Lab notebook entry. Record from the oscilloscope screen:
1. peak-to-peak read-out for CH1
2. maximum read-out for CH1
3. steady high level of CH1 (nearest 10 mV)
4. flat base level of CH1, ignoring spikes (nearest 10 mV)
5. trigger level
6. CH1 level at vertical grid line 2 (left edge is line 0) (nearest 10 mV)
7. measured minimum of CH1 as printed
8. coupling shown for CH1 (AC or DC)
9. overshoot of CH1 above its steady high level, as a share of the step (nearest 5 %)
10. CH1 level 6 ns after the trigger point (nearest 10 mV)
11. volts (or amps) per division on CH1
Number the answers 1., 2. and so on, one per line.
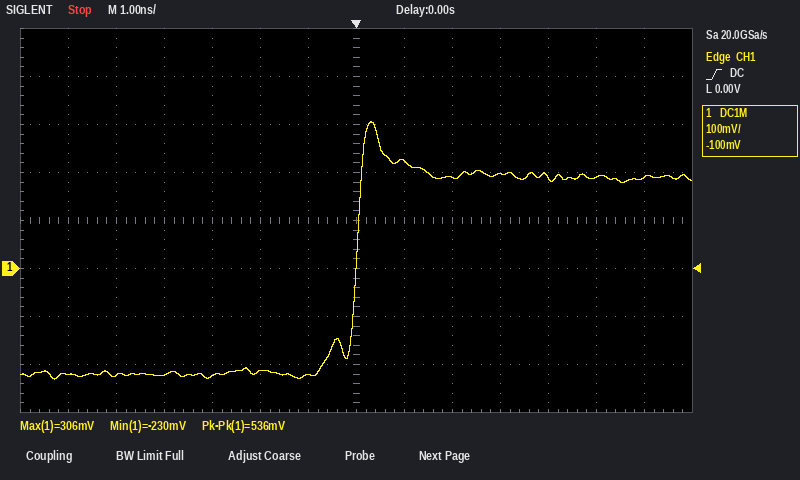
1. 536 mV
2. 306 mV
3. 190 mV
4. -220 mV
5. 0.00 V
6. -220 mV
7. -230 mV
8. DC
9. 30 %
10. 190 mV
11. 100 mV
